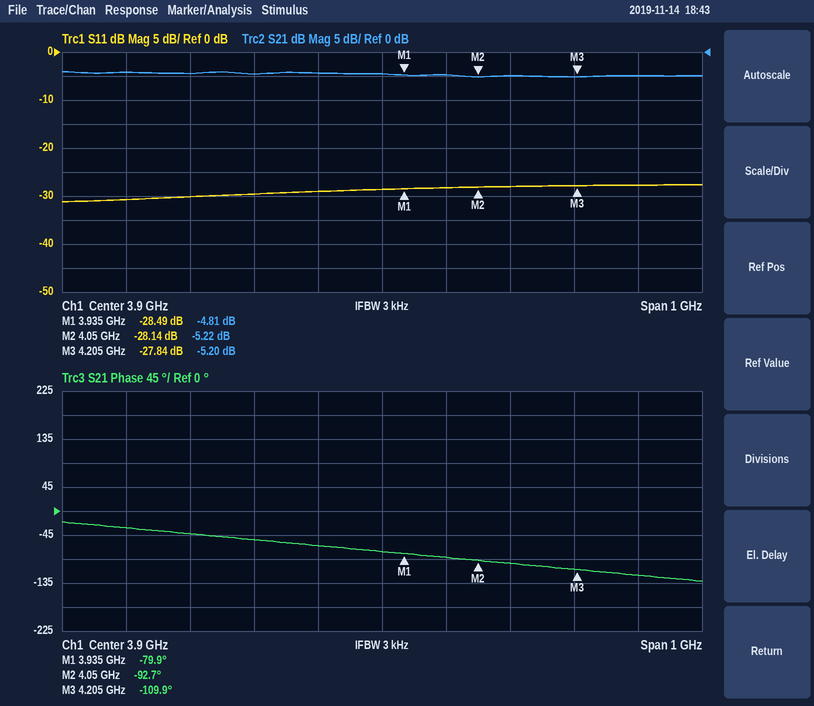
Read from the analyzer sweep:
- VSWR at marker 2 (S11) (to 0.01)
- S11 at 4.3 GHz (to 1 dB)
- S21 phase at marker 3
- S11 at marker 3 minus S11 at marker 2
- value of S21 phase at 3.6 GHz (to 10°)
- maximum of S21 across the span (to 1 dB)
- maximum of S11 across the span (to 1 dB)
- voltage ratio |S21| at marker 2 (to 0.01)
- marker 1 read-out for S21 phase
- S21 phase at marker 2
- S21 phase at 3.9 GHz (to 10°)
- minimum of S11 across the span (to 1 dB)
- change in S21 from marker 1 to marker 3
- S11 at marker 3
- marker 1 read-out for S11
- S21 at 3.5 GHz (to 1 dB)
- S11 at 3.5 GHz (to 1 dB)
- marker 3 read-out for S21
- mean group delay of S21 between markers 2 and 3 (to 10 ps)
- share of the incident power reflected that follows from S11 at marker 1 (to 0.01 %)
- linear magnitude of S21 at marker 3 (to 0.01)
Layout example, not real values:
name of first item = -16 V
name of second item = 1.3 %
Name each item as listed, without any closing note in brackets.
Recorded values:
VSWR at marker 2 (S11) = 1.08
S11 at 4.3 GHz = -28 dB
S21 phase at marker 3 = -109.9°
S11 at marker 3 minus S11 at marker 2 = 0.30 dB
value of S21 phase at 3.6 GHz = -40°
maximum of S21 across the span = -4 dB
maximum of S11 across the span = -28 dB
voltage ratio |S21| at marker 2 = 0.55
marker 1 read-out for S21 phase = -79.9°
S21 phase at marker 2 = -92.7°
S21 phase at 3.9 GHz = -80°
minimum of S11 across the span = -31 dB
change in S21 from marker 1 to marker 3 = -0.39 dB
S11 at marker 3 = -27.84 dB
marker 1 read-out for S11 = -28.49 dB
S21 at 3.5 GHz = -4 dB
S11 at 3.5 GHz = -31 dB
marker 3 read-out for S21 = -5.20 dB
mean group delay of S21 between markers 2 and 3 = 310 ps
share of the incident power reflected that follows from S11 at marker 1 = 0.14 %
linear magnitude of S21 at marker 3 = 0.55
